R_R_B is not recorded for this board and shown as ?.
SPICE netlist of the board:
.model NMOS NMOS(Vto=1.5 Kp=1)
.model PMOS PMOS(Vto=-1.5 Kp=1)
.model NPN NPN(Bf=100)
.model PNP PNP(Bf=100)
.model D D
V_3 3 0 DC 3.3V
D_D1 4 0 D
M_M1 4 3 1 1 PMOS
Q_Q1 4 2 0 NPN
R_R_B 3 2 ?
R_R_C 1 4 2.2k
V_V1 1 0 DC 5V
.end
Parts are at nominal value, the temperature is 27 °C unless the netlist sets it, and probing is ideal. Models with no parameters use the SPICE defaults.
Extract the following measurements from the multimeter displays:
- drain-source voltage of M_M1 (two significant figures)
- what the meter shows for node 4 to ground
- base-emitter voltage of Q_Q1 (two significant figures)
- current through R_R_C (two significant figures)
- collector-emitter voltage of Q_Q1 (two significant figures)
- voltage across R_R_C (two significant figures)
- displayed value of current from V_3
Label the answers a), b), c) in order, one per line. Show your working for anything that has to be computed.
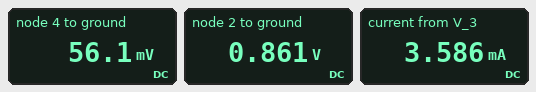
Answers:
a) 56.1 mV - 5 V = -4.9 V
b) 56.1 mV
c) 861 mV = 860 mV
d) (5 V - 56.1 mV) / 2.2 kΩ = 2.2 mA
e) 56.1 mV = 56 mV
f) 5 V - 56.1 mV = 4.9 V
g) 3.586 mA
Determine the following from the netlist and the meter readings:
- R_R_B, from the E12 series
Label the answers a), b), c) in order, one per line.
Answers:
a) 680 Ω
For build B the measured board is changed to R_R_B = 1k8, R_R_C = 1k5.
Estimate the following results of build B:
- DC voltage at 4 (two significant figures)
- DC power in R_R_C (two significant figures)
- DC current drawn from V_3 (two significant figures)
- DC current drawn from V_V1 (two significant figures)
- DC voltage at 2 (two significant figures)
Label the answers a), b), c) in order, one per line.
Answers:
a) 81 mV
b) 16 mW
c) 1.4 mA
d) 23 mA
e) 860 mV
